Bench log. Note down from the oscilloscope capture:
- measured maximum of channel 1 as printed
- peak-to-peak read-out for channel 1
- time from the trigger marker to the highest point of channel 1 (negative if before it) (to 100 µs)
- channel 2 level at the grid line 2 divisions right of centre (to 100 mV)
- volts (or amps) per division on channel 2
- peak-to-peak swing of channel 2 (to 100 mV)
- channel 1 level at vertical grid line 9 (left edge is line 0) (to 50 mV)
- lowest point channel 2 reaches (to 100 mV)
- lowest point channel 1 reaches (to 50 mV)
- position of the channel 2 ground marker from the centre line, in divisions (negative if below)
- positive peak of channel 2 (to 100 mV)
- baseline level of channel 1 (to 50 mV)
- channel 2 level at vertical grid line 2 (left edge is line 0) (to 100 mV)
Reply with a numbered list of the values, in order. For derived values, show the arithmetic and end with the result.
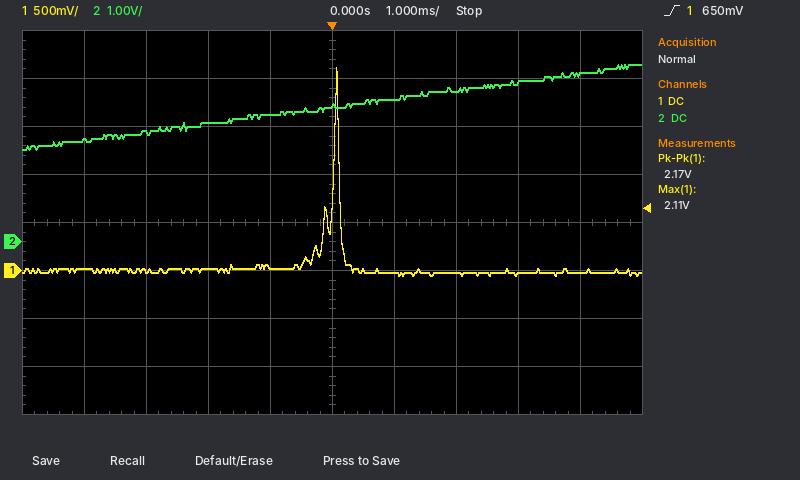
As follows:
1. 2.11 V
2. 2.17 V
3. +100 µs
4. 3.1 V
5. 1 V
6. 3.7 V − (1.9 V) = 1.8 V
7. 0 mV
8. 1.9 V
9. -50 mV
10. -0.4 div
11. 3.7 V
12. 0 mV
13. 2.3 V
